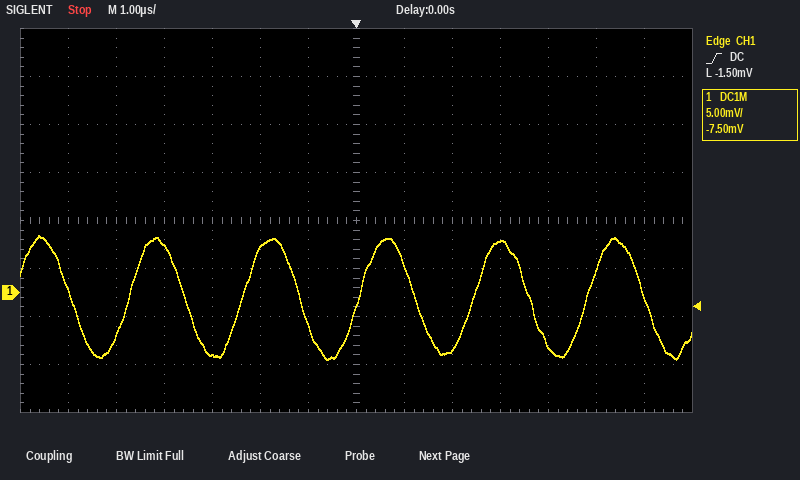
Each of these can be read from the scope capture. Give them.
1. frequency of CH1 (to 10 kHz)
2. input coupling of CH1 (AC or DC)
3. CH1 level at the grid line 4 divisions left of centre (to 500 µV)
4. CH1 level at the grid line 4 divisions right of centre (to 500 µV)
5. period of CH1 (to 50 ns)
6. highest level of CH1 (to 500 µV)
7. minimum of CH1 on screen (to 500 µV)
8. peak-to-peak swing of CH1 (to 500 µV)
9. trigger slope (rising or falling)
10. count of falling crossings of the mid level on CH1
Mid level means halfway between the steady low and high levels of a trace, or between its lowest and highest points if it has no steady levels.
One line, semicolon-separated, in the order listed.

420 kHz; DC; 5.0 mV; -5.5 mV; 2.40 µs; 6.0 mV; -7.0 mV; 13.0 mV; rising; 6
